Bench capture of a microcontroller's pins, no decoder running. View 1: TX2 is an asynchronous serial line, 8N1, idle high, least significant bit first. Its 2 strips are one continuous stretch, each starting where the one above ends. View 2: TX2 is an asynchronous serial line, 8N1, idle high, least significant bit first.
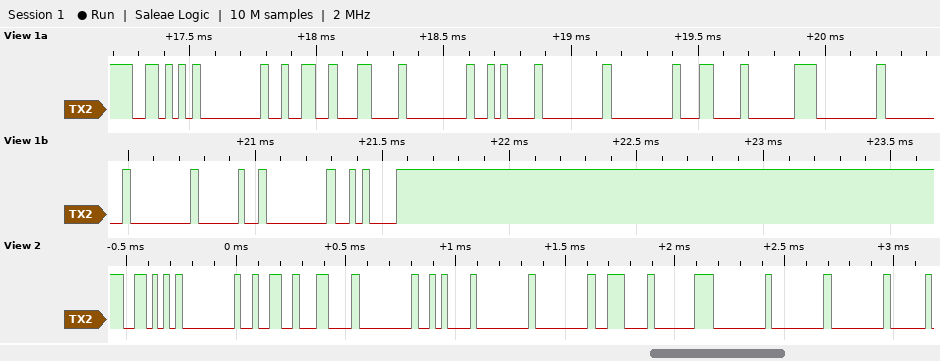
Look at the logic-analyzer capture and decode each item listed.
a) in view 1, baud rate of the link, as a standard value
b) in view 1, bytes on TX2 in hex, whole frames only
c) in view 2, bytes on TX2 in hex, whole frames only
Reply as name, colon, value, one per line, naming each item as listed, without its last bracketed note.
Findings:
in view 1, baud rate of the link, as a standard value: 38400 baud
in view 1, bytes on TX2 in hex, whole frames only: 0x56 0x00 0x32 0x0C 0x00 0x0A 0x00 0x00 0x0C 0xC0 0x00 0x00 0x00 0x20 0x00 0x0A
in view 2, bytes on TX2 in hex, whole frames only: 0x56 0x00 0x32 0x0C 0x00 0x0A 0x00 0x00 0x0E 0xC0 0x00 0x00 0x00
